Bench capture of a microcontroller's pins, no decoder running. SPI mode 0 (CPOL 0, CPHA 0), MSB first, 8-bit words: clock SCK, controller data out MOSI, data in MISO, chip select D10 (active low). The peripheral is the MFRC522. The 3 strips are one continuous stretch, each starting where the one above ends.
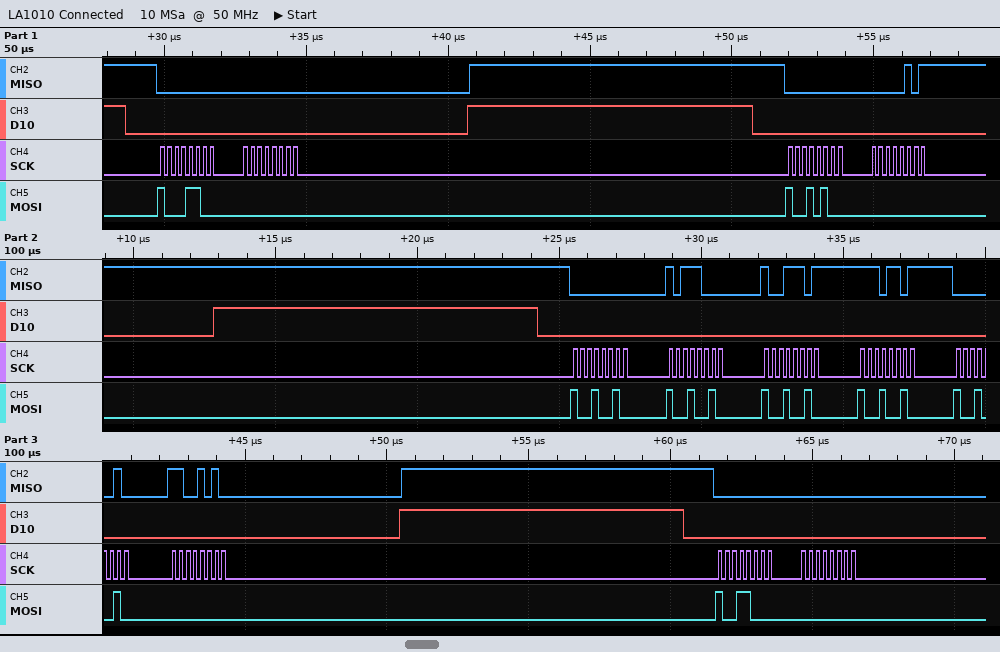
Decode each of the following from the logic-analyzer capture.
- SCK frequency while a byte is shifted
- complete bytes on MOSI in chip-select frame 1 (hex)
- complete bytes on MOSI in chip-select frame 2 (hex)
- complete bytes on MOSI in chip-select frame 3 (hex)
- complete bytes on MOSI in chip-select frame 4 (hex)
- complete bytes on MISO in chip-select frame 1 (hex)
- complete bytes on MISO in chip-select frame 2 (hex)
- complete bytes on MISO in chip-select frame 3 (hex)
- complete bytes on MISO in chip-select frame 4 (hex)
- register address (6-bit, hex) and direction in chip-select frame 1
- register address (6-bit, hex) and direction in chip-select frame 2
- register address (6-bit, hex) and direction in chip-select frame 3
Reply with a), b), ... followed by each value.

a) 4 MHz
b) 8C 00
c) 94 00
d) 92 92 92 92 92 00
e) 98 00
f) 00 00
g) 00 05
h) 00 B8 9D ED 02 CA
i) 00 00
j) 0x06 read
k) 0x0A read
l) 0x09 read
